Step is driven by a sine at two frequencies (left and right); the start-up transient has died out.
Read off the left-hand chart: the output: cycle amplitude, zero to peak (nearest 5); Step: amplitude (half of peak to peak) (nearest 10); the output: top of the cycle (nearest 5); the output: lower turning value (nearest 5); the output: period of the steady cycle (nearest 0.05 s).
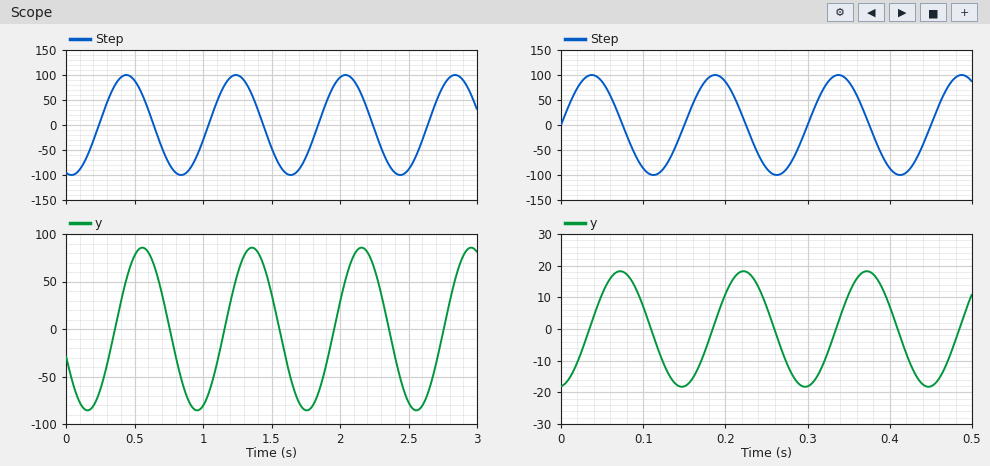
85
100
85
-85
0.80 s
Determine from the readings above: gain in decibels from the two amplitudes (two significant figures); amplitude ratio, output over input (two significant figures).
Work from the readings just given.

-1.4 dB
0.85
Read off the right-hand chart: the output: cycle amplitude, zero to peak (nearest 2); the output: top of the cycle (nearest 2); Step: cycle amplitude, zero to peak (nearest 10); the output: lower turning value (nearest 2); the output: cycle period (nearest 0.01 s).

18
18
100
-18
0.15 s
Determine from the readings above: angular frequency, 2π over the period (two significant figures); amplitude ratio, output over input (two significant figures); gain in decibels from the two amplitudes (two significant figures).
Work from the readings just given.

42 rad/s
0.18
-15 dB
